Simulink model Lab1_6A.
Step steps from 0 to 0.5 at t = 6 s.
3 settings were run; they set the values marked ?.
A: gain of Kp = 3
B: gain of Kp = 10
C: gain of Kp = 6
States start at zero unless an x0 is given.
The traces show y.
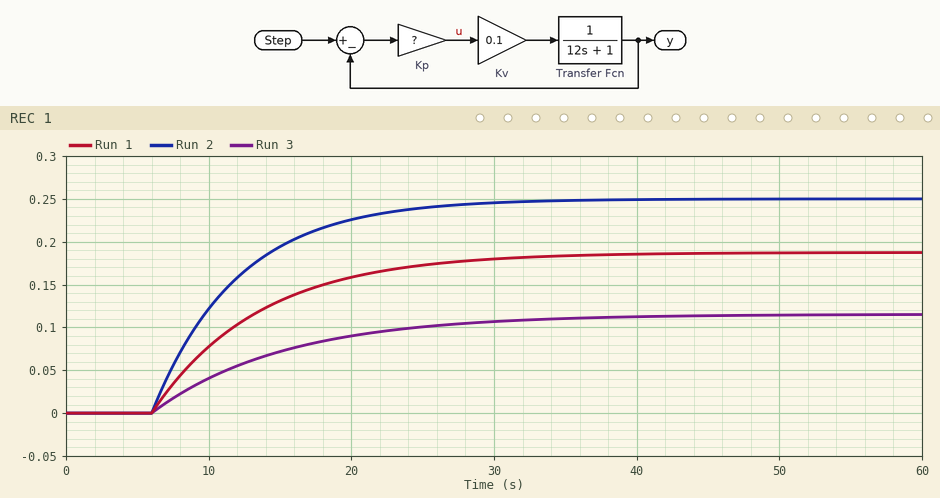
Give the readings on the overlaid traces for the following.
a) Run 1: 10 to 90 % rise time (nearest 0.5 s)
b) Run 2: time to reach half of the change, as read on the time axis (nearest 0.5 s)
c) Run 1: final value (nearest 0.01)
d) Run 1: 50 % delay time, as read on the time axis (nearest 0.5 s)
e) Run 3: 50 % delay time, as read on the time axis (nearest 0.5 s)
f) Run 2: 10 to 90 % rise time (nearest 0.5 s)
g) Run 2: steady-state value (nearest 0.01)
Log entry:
16.5 s
10.0 s
0.19
11.0 s
12.5 s
13.0 s
0.25
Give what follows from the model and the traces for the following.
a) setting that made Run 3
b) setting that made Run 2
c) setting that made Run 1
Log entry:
A
B
C
